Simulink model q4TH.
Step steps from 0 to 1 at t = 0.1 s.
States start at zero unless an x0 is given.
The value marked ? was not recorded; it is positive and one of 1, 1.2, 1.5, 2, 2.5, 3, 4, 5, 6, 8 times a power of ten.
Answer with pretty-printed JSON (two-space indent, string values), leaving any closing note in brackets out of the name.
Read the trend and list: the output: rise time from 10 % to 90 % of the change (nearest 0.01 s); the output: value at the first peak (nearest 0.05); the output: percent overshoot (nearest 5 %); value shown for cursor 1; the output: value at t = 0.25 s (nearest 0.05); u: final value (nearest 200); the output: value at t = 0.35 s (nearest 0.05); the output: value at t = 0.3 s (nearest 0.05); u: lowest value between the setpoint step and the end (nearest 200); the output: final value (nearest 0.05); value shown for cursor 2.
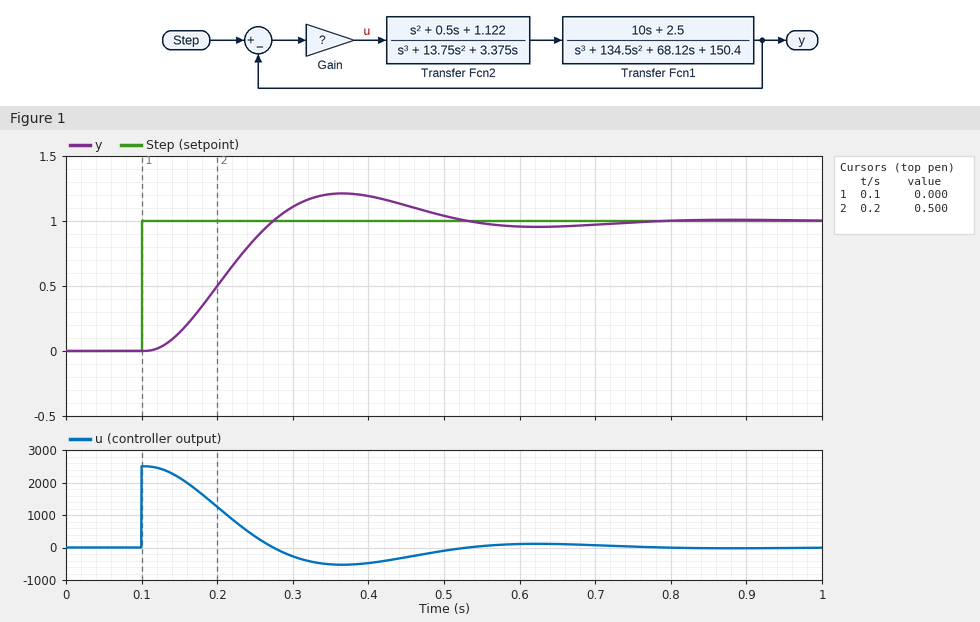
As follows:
{
  "the output: rise time from 10 % to 90 % of the change": "0.11 s",
  "the output: value at the first peak": "1.20",
  "the output: percent overshoot": "20 %",
  "value shown for cursor 1": "0.000",
  "the output: value at t = 0.25 s": "0.85",
  "u: final value": "0",
  "the output: value at t = 0.35 s": "1.20",
  "the output: value at t = 0.3 s": "1.10",
  "u: lowest value between the setpoint step and the end": "-600",
  "the output: final value": "1.00",
  "value shown for cursor 2": "0.500"
}
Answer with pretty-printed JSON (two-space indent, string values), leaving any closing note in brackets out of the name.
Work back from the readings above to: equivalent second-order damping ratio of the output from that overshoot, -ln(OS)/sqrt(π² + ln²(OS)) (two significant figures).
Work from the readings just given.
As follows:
{
  "equivalent second-order damping ratio of the output from that overshoot, -ln(OS)/sqrt(π² + ln²(OS))": "0.46"
}
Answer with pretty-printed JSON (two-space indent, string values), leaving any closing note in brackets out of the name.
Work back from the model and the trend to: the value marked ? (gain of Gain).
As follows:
{
  "the value marked ?": "2500"
}
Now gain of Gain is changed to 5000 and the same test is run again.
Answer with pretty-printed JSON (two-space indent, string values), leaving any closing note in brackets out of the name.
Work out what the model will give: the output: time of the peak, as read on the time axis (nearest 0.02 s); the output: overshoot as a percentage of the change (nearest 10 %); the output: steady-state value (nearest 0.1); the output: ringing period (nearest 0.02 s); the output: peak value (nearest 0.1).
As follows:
{
  "the output: time of the peak, as read on the time axis": "0.28 s",
  "the output: overshoot as a percentage of the change": "40 %",
  "the output: steady-state value": "1.0",
  "the output: ringing period": "0.34 s",
  "the output: peak value": "1.4"
}
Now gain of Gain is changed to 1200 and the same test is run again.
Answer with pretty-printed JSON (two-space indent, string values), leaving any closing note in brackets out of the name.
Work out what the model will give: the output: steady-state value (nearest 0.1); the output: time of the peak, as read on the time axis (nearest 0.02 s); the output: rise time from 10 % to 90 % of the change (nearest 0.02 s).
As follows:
{
  "the output: steady-state value": "1.0",
  "the output: time of the peak, as read on the time axis": "0.56 s",
  "the output: rise time from 10 % to 90 % of the change": "0.22 s"
}
